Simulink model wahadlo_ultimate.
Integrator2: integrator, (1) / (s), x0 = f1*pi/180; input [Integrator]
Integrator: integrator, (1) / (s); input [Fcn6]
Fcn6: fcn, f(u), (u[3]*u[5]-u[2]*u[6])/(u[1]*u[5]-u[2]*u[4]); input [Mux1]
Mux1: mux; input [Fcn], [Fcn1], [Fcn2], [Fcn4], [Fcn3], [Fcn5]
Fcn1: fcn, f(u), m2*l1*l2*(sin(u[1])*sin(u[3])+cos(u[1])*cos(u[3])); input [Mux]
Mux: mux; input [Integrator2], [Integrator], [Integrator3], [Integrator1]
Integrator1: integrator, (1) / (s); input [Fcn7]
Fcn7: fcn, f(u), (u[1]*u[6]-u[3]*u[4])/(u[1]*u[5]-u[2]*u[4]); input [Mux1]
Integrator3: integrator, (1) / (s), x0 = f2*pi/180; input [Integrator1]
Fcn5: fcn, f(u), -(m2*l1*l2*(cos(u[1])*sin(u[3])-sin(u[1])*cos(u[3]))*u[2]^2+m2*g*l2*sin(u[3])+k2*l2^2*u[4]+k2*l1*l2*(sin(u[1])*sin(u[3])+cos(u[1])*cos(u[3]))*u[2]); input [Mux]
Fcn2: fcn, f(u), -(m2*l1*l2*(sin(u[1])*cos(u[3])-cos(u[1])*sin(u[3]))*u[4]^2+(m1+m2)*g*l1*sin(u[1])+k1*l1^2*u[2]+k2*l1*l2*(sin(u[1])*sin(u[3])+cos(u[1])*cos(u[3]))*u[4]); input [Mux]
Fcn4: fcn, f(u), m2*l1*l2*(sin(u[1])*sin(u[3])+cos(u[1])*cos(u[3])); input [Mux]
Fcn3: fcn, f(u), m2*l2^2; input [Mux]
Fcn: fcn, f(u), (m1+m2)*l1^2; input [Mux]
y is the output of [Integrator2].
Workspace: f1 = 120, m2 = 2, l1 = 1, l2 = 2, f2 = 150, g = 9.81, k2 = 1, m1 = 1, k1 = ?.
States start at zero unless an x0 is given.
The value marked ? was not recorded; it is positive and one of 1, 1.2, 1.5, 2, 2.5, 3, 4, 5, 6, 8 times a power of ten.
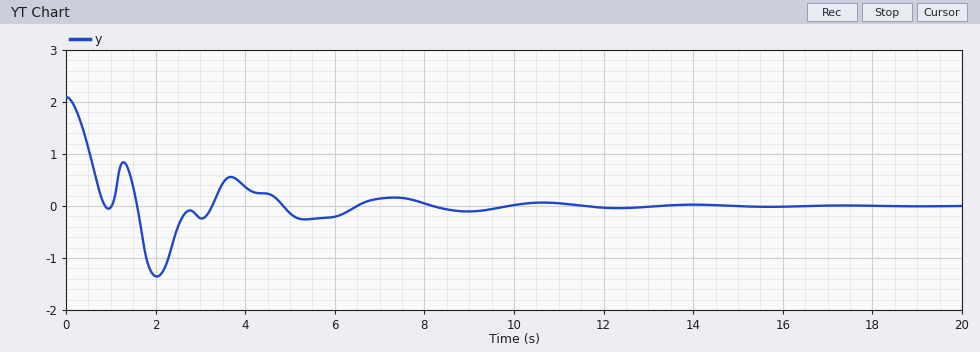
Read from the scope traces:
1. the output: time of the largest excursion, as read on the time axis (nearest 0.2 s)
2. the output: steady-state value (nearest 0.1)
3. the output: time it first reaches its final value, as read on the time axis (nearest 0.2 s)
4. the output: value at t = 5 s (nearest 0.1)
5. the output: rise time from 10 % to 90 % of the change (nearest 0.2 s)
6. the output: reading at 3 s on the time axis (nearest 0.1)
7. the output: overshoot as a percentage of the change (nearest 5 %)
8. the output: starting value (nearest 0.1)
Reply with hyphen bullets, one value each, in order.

- 2.0 s
- 0.0
- 0.8 s
- -0.1
- 0.6 s
- -0.2
- 65 %
- 2.1
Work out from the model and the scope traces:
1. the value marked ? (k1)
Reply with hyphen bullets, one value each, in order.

- 3
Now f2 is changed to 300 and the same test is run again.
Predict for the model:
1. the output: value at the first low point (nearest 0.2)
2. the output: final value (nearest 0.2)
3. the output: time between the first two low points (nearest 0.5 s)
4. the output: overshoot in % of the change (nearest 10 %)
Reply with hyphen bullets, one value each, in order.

- -1.0
- 0.0
- 1.5 s
- 50 %
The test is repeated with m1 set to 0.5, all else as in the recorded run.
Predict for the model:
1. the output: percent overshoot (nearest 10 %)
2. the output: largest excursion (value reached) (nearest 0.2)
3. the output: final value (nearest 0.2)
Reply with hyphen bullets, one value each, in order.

- 50 %
- -1.0
- 0.0
